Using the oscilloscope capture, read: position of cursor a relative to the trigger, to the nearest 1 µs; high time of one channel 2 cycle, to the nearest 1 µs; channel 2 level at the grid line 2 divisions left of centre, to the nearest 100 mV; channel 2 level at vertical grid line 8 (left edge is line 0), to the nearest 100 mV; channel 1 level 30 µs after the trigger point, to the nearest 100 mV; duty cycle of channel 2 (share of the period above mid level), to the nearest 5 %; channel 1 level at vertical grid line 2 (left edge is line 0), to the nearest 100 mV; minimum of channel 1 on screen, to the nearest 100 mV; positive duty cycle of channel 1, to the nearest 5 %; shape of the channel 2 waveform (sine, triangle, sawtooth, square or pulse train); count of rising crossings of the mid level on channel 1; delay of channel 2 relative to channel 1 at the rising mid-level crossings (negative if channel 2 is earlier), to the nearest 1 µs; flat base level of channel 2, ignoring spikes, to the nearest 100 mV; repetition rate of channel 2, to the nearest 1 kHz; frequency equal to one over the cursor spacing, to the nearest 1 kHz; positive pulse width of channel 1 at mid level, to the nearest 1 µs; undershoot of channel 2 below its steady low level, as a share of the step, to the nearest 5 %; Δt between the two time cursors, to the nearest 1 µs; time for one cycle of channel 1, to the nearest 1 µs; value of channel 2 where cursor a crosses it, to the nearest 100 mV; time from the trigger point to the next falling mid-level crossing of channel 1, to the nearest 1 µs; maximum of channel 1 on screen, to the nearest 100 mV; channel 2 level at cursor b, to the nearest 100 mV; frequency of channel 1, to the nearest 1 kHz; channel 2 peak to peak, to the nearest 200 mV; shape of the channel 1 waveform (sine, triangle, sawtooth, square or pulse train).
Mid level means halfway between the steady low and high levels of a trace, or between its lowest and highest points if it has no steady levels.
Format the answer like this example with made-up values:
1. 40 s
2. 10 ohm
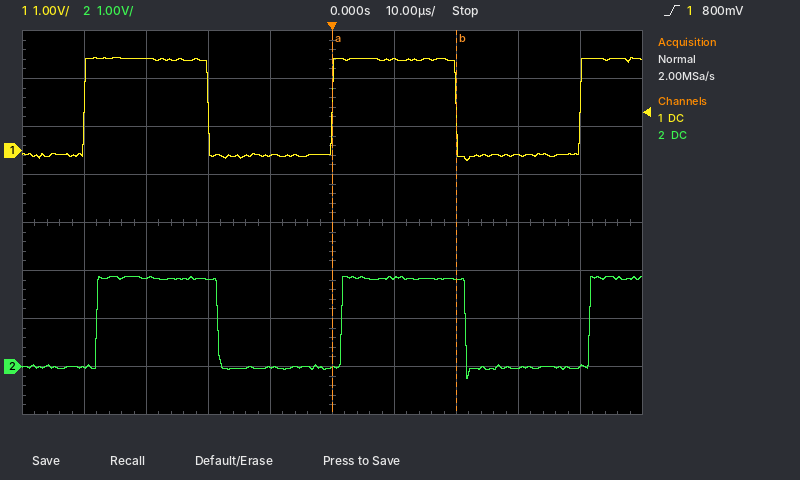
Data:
1. 0 µs
2. 20 µs
3. 1.8 V
4. 0.0 V
5. -100 mV
6. 50 %
7. 1.9 V
8. -200 mV
9. 50 %
10. square
11. 3
12. +2 µs
13. 0.0 V
14. 25 kHz
15. 50 kHz
16. 20 µs
17. 10 %
18. 20 µs
19. 40 µs
20. 0.0 V
21. 20 µs
22. 1.9 V
23. 1.8 V
24. 25 kHz
25. 2.2 V
26. square
